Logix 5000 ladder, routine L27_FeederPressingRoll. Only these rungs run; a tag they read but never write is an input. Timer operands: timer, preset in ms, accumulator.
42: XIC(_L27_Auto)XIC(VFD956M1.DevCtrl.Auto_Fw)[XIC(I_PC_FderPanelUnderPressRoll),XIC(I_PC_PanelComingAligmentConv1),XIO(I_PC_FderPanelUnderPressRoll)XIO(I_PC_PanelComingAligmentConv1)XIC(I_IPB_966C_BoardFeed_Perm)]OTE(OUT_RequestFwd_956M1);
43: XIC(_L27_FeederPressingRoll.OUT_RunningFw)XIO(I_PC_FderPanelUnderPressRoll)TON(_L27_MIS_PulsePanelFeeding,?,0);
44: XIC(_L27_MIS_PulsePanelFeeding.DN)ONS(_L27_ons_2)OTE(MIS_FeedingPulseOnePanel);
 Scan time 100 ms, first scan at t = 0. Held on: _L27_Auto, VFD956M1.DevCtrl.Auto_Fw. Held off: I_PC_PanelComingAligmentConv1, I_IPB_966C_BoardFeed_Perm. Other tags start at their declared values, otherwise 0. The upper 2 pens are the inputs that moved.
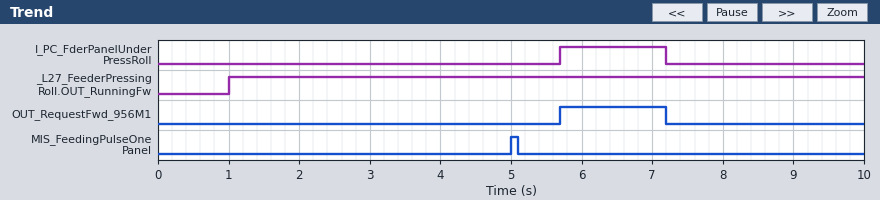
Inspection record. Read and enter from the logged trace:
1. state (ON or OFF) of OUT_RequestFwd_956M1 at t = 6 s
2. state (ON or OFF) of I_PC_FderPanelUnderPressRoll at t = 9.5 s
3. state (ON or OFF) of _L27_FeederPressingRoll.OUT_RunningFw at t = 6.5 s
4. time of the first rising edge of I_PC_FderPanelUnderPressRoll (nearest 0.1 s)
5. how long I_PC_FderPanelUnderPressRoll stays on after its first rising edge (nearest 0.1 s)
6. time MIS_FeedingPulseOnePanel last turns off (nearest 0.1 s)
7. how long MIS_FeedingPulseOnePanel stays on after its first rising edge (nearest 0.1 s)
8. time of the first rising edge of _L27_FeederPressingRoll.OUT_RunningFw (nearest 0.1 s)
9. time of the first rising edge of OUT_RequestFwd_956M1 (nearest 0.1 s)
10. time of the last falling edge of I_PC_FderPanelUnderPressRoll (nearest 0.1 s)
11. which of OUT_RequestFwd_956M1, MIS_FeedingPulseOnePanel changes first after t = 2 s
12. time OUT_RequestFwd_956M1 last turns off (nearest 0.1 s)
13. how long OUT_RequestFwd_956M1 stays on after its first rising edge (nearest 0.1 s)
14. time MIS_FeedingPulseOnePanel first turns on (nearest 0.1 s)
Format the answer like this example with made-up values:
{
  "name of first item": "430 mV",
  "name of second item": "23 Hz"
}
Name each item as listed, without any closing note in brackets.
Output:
{
  "state (ON or OFF) of OUT_RequestFwd_956M1 at t = 6 s": "ON",
  "state (ON or OFF) of I_PC_FderPanelUnderPressRoll at t = 9.5 s": "OFF",
  "state (ON or OFF) of _L27_FeederPressingRoll.OUT_RunningFw at t = 6.5 s": "ON",
  "time of the first rising edge of I_PC_FderPanelUnderPressRoll": "5.7 s",
  "how long I_PC_FderPanelUnderPressRoll stays on after its first rising edge": "1.5 s",
  "time MIS_FeedingPulseOnePanel last turns off": "5.1 s",
  "how long MIS_FeedingPulseOnePanel stays on after its first rising edge": "0.1 s",
  "time of the first rising edge of _L27_FeederPressingRoll.OUT_RunningFw": "1.0 s",
  "time of the first rising edge of OUT_RequestFwd_956M1": "5.7 s",
  "time of the last falling edge of I_PC_FderPanelUnderPressRoll": "7.2 s",
  "which of OUT_RequestFwd_956M1, MIS_FeedingPulseOnePanel changes first after t = 2 s": "MIS_FeedingPulseOnePanel",
  "time OUT_RequestFwd_956M1 last turns off": "7.2 s",
  "how long OUT_RequestFwd_956M1 stays on after its first rising edge": "1.5 s",
  "time MIS_FeedingPulseOnePanel first turns on": "5.0 s"
}
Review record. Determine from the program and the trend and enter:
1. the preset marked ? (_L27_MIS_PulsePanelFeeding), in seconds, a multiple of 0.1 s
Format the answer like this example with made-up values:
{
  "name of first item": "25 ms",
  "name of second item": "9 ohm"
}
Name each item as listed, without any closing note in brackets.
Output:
{
  "the preset marked ? (_L27_MIS_PulsePanelFeeding), in seconds, a multiple of 0.1 s": "4.0 s"
}
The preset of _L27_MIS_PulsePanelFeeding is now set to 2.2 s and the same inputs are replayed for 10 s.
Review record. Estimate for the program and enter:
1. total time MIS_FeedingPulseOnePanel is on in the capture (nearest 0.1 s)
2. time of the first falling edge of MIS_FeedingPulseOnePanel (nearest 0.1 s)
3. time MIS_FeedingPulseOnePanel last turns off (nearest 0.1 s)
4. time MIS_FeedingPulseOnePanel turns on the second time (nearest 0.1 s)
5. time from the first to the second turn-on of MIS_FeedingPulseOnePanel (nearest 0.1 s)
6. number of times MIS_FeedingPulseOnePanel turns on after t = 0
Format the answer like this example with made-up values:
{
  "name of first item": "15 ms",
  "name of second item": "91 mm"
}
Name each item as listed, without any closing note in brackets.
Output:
{
  "total time MIS_FeedingPulseOnePanel is on in the capture": "0.2 s",
  "time of the first falling edge of MIS_FeedingPulseOnePanel": "3.3 s",
  "time MIS_FeedingPulseOnePanel last turns off": "9.5 s",
  "time MIS_FeedingPulseOnePanel turns on the second time": "9.4 s",
  "time from the first to the second turn-on of MIS_FeedingPulseOnePanel": "6.2 s",
  "number of times MIS_FeedingPulseOnePanel turns on after t = 0": "2"
}
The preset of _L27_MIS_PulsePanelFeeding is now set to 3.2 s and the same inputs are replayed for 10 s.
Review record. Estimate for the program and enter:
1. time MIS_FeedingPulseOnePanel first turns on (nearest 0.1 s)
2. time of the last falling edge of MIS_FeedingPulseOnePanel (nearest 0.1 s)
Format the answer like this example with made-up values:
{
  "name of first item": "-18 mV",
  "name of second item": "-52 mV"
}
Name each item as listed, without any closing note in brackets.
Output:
{
  "time MIS_FeedingPulseOnePanel first turns on": "4.2 s",
  "time of the last falling edge of MIS_FeedingPulseOnePanel": "4.3 s"
}
